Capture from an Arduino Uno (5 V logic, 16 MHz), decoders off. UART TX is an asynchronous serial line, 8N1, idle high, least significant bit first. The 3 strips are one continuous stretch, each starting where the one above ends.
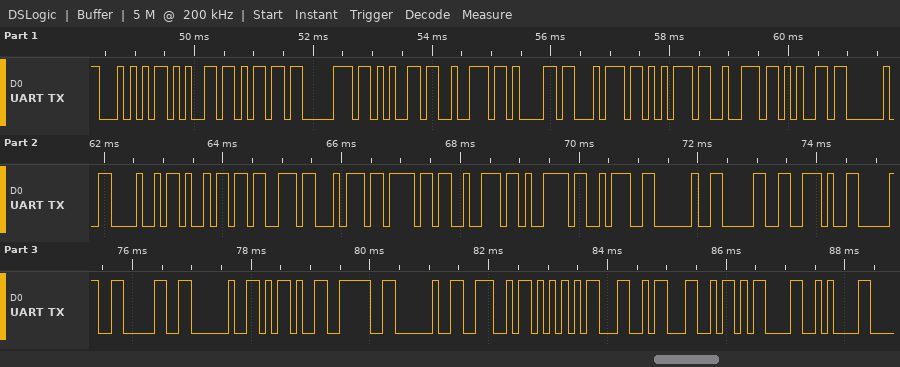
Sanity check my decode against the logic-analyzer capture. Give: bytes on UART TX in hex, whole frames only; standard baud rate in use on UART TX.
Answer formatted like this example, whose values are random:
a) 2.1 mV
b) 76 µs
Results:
a) 0x54 0x65 0x6D 0x70 0x65 0x72 0x61 0x74 0x75 0x72 0x65 0x20 0x48 0x69 0x73 0x74 0x6F 0x72 0x79 0x3A 0x20 0x30 0x2E 0x30 0x30 0x20 0x2D 0x3E 0x20 0x4E 0x55 0x4C 0x4C 0x0D 0x0A
b) 9600 baud
